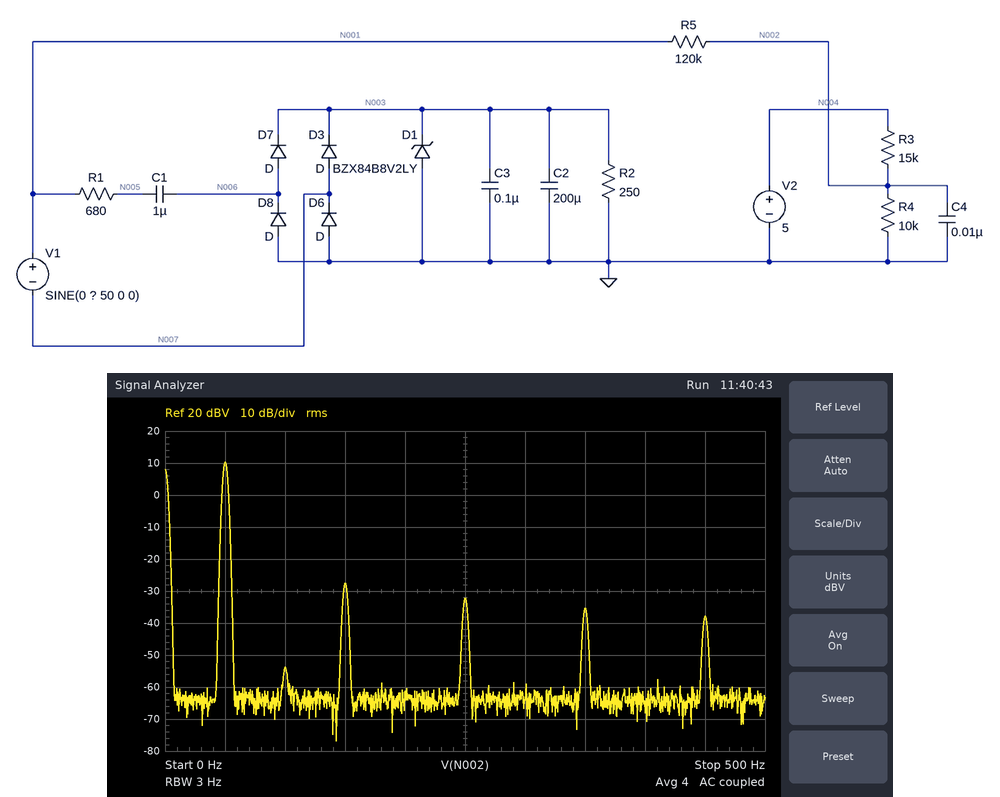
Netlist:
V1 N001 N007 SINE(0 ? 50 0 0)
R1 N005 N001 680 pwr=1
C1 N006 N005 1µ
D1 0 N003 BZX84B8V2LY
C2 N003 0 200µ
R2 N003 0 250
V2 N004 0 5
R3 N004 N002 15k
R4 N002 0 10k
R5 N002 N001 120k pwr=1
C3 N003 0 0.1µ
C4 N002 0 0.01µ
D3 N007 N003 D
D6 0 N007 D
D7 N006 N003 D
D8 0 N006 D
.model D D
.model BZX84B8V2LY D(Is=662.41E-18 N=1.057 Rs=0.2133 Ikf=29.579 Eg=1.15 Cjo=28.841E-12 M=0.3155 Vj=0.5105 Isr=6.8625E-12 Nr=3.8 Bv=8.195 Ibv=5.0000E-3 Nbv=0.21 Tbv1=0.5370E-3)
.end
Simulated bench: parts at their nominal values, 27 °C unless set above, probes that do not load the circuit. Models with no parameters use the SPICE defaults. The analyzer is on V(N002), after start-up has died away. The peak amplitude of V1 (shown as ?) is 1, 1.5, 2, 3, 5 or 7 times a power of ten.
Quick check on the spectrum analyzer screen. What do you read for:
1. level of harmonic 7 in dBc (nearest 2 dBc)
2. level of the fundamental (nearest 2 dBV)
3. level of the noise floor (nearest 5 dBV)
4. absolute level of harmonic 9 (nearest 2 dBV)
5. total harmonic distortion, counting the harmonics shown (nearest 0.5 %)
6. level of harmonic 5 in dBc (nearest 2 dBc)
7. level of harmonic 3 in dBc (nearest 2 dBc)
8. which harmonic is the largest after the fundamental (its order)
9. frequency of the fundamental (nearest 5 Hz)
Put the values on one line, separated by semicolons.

-46 dBc; 10 dBV; -65 dBV; -38 dBV; 1.5 %; -42 dBc; -38 dBc; 3; 50 Hz
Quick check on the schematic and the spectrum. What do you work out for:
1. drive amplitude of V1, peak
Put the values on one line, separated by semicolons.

100 V
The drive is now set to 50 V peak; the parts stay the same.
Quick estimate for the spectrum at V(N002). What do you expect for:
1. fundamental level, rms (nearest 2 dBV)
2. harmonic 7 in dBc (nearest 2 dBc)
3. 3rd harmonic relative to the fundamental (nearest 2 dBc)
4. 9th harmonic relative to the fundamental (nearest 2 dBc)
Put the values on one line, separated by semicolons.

4 dBV; -44 dBc; -36 dBc; -46 dBc
